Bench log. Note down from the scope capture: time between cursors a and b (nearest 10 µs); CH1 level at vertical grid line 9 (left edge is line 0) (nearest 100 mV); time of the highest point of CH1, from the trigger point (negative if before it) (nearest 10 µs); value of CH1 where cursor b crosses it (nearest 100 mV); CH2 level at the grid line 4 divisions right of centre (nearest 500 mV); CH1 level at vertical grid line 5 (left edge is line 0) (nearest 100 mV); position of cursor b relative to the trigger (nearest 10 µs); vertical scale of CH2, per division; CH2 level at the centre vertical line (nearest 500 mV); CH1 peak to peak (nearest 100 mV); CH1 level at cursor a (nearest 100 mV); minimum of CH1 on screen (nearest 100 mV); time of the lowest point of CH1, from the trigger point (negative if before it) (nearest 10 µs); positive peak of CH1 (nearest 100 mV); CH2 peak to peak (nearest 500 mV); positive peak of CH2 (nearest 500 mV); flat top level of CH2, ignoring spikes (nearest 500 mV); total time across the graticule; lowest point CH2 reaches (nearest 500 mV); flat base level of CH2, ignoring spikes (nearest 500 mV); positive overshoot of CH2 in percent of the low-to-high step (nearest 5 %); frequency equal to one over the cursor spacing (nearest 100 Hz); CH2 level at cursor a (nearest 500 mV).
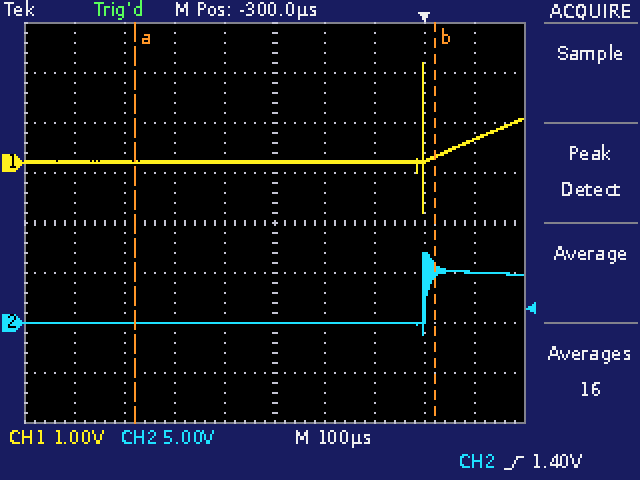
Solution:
600 µs
500 mV
0 µs
100 mV
5.0 V
0.0 V
+20 µs
5 V
0.0 V
3.0 V
0.0 V
-1.0 V
0 µs
2.0 V
8.0 V
7.0 V
5.0 V
1 ms
-1.0 V
0.0 V
40 %
1.7 kHz
0.0 V
